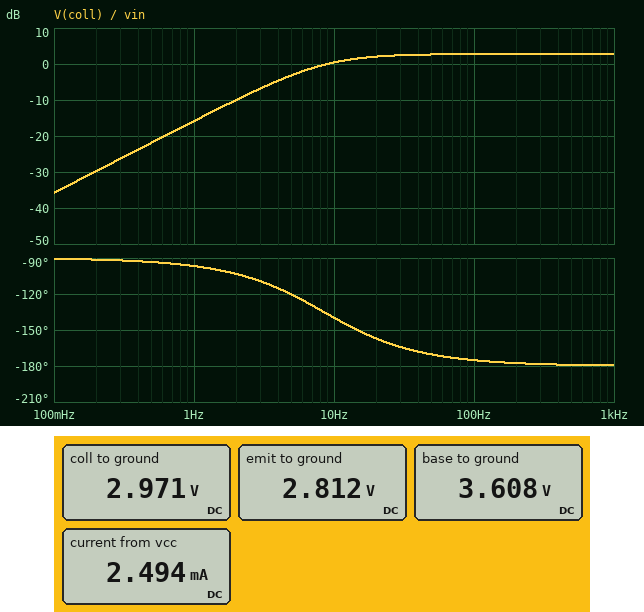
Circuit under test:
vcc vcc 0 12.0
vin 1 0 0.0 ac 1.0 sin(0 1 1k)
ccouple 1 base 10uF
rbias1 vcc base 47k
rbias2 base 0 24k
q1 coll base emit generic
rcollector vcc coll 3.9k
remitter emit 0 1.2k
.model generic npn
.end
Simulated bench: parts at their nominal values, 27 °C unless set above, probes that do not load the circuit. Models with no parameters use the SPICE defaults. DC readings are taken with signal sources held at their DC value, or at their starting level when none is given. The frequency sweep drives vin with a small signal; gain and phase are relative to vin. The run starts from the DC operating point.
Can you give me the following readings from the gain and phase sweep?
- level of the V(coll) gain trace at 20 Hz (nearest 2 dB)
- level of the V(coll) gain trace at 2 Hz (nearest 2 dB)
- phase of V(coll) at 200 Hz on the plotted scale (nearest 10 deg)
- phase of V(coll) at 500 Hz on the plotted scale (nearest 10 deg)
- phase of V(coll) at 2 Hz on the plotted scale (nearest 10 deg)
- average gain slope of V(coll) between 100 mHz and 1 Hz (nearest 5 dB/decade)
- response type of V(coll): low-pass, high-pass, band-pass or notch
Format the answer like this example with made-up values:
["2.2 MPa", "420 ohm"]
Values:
["2 dB", "-10 dB", "-180 deg", "-180 deg", "-100 deg", "20 dB/decade", "high-pass"]
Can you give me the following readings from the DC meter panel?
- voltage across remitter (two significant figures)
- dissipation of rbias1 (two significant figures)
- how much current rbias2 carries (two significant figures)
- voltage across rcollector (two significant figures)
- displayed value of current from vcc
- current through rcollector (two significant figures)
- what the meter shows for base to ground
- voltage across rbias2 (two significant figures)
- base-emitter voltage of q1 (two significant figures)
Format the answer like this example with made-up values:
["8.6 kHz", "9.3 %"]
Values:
["2.8 V", "1.5 mW", "150 µA", "9.0 V", "2.494 mA", "2.3 mA", "3.608 V", "3.6 V", "800 mV"]
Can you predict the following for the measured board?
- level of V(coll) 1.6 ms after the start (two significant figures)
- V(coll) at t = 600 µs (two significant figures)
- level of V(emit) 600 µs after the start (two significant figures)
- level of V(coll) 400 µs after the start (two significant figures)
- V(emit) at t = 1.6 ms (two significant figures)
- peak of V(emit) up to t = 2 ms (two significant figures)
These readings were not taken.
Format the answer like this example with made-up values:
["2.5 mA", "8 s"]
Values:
["5.0 V", "4.9 V", "2.2 V", "3.4 V", "2.2 V", "3.8 V"]
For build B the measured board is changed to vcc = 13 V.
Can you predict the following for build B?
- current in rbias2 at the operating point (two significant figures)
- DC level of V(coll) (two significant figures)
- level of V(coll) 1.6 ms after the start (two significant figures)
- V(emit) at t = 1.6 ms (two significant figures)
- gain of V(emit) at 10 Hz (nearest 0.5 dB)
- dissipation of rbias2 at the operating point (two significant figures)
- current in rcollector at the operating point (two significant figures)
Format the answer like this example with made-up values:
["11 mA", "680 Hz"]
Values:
["160 µA", "3.2 V", "5.2 V", "2.4 V", "-3.5 dB", "620 µW", "2.5 mA"]
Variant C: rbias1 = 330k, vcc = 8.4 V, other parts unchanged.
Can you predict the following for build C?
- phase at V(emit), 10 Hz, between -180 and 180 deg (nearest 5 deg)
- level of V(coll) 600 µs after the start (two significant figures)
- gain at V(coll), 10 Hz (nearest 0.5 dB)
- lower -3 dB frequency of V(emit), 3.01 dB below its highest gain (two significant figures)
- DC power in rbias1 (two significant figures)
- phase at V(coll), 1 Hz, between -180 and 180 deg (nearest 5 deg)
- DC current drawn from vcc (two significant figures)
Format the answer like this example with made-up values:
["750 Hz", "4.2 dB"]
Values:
["5 deg", "8.4 V", "-25.5 dB", "710 mHz", "190 µW", "-145 deg", "24 µA"]
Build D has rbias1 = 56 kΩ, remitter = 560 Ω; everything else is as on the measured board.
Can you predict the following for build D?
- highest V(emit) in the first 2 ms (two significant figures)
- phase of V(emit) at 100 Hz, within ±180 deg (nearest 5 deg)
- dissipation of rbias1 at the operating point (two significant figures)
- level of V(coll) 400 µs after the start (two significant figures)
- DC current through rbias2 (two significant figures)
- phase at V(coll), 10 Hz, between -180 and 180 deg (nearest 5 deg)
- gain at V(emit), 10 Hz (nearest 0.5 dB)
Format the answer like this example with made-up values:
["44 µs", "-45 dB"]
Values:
["2.5 V", "15 deg", "1.7 mW", "2.1 V", "97 µA", "70 deg", "-10.0 dB"]
